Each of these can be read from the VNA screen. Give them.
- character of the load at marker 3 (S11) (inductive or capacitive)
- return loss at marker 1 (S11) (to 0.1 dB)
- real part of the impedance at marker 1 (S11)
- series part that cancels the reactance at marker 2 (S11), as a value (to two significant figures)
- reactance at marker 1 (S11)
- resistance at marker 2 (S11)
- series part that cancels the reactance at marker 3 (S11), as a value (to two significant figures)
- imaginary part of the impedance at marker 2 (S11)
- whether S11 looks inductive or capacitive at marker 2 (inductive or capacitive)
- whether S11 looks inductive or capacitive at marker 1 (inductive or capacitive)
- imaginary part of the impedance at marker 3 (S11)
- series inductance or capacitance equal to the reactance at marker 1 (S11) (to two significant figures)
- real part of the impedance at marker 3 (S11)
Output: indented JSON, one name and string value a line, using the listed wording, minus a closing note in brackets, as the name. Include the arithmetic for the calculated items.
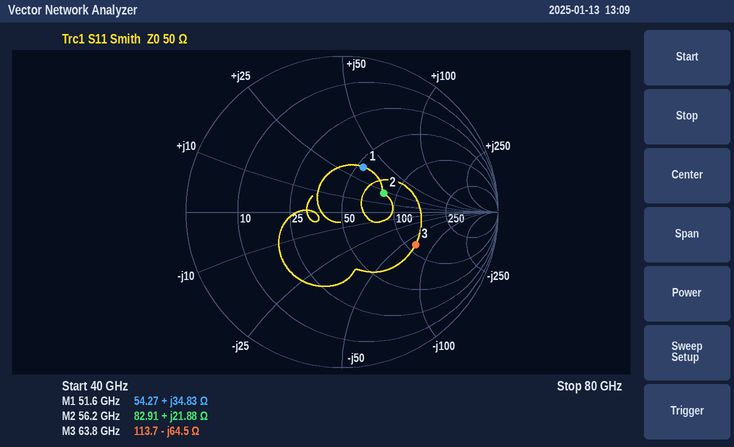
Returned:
{
  "character of the load at marker 3 (S11)": "capacitive",
  "return loss at marker 1 (S11)": "9.9 dB",
  "real part of the impedance at marker 1": "54.27 Ω",
  "series part that cancels the reactance at marker 2 (S11), as a value": "C = 1/(2π × 56.2 GHz × 21.88 Ω) ≈ 129 fF, so 130 fF to two significant figures",
  "reactance at marker 1": "+34.83 Ω",
  "resistance at marker 2": "82.91 Ω",
  "series part that cancels the reactance at marker 3 (S11), as a value": "L = 64.5 Ω/(2π × 63.8 GHz) ≈ 161 pH, so 160 pH to two significant figures",
  "imaginary part of the impedance at marker 2": "+21.88 Ω",
  "whether S11 looks inductive or capacitive at marker 2": "inductive",
  "whether S11 looks inductive or capacitive at marker 1": "inductive",
  "imaginary part of the impedance at marker 3": "-64.5 Ω",
  "series inductance or capacitance equal to the reactance at marker 1 (S11)": "L = 34.83 Ω/(2π × 51.6 GHz) ≈ 107 pH, so 110 pH to two significant figures",
  "real part of the impedance at marker 3": "113.7 Ω"
}
